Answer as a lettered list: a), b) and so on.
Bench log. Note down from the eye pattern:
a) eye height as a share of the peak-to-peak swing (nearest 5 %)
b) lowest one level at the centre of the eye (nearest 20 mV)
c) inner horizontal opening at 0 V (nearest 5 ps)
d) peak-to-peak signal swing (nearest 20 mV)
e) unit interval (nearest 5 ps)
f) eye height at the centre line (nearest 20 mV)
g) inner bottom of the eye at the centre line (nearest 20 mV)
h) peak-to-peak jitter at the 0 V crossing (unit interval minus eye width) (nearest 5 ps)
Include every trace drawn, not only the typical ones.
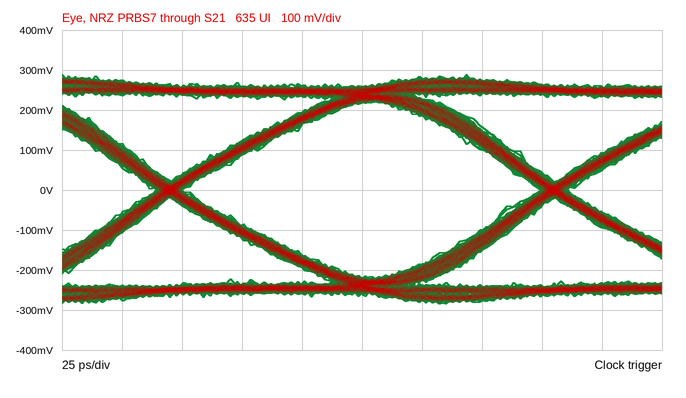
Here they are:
a) 75 %
b) 220 mV
c) 150 ps
d) 580 mV
e) 160 ps
f) 440 mV
g) -220 mV
h) 10 ps
